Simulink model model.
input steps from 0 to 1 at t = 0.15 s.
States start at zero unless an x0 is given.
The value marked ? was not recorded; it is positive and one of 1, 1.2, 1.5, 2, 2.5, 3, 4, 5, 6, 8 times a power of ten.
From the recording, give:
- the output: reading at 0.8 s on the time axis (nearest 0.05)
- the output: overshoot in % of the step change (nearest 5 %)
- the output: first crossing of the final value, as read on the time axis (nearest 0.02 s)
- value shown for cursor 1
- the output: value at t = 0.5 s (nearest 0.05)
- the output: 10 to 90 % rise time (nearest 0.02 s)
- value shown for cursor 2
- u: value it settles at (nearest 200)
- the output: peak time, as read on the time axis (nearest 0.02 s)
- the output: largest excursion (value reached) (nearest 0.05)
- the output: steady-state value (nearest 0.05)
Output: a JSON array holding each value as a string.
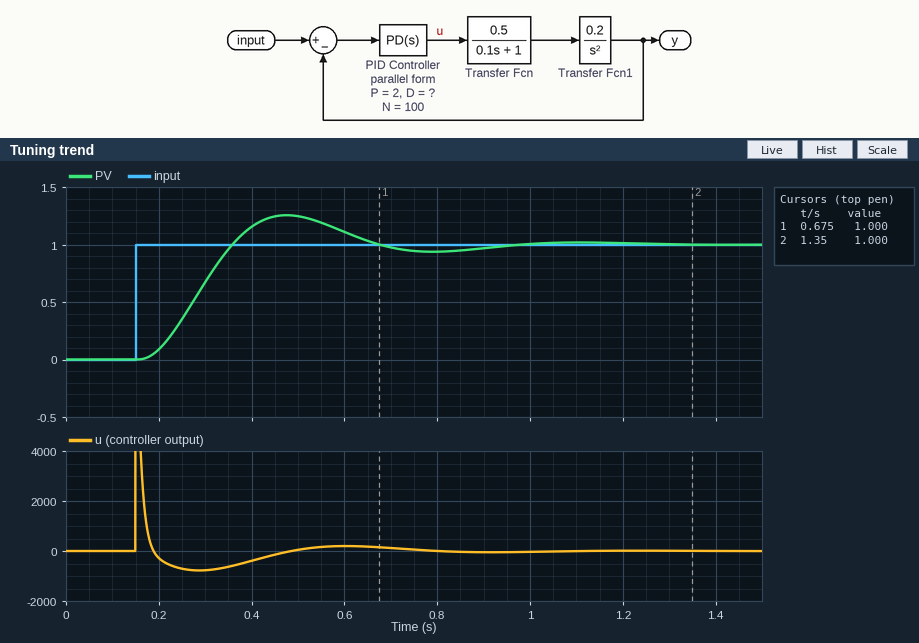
["0.95", "25 %", "0.36 s", "1.000", "1.25", "0.14 s", "1.000", "0", "0.48 s", "1.25", "1.00"]
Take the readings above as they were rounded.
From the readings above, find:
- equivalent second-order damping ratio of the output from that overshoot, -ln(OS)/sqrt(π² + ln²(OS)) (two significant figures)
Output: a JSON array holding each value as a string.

["0.40"]
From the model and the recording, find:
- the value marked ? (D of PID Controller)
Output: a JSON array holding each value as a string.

["120"]
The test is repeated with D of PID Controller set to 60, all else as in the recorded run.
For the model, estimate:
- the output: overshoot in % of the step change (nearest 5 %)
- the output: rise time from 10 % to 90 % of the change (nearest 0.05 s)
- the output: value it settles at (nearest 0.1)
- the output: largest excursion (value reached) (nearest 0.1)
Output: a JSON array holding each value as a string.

["10 %", "0.25 s", "1.0", "1.1"]
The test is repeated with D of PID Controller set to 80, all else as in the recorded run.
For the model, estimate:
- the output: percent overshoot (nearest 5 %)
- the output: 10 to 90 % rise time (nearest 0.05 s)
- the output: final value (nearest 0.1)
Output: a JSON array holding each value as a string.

["15 %", "0.20 s", "1.0"]
